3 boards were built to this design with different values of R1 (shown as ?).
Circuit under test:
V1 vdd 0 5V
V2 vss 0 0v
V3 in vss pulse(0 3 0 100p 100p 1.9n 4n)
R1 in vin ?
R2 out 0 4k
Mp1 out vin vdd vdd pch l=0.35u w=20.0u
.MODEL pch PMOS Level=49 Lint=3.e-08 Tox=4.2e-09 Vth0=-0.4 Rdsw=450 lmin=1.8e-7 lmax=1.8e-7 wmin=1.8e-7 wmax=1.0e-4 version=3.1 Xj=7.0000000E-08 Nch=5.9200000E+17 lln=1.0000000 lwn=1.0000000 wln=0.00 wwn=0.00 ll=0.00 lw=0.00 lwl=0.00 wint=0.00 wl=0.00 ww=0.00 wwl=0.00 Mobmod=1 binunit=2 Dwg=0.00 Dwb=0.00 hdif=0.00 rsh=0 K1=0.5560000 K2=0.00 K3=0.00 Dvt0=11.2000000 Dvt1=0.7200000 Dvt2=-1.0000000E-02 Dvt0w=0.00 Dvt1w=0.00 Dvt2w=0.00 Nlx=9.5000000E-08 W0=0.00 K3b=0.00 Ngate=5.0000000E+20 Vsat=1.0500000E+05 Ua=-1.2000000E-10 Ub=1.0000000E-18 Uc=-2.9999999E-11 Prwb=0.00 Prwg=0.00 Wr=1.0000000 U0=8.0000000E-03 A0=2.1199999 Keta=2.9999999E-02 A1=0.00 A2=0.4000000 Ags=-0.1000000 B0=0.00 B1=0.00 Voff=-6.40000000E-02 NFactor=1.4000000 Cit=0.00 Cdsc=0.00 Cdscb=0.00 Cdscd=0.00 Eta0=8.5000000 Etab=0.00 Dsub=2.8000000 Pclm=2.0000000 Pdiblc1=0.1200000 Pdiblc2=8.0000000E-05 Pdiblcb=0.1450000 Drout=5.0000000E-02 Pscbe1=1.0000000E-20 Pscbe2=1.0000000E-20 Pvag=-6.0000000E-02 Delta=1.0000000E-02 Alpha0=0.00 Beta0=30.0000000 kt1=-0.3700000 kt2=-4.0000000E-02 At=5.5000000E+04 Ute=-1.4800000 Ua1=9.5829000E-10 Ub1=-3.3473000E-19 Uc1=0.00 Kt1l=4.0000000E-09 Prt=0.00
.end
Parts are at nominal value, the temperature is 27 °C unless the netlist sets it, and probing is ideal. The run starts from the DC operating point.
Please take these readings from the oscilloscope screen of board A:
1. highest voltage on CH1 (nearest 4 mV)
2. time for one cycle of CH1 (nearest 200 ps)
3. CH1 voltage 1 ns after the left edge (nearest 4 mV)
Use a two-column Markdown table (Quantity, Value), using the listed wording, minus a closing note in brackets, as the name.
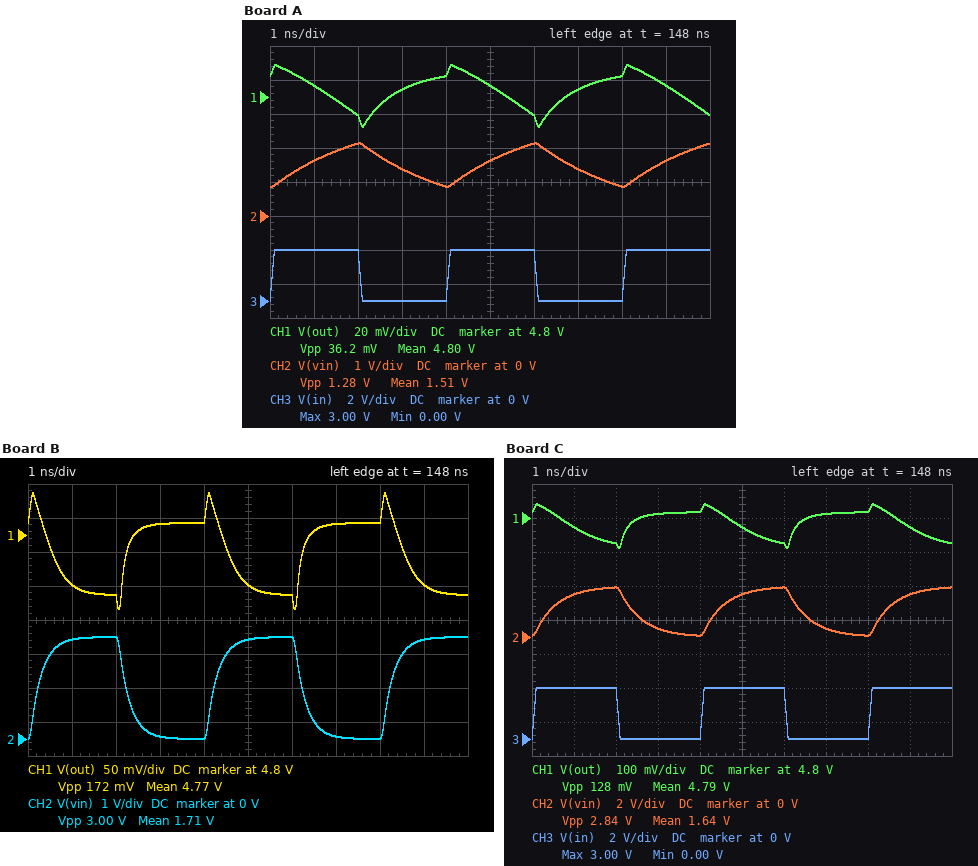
| Quantity | Value |
|---|---|
| highest voltage on CH1 | 4.820 V |
| time for one cycle of CH1 | 4.0 ns |
| CH1 voltage 1 ns after the left edge | 4.808 V |
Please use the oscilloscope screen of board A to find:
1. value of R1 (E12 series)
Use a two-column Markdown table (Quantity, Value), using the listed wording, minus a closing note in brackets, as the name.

| Quantity | Value |
|---|---|
| value of R1 | 33 kΩ |
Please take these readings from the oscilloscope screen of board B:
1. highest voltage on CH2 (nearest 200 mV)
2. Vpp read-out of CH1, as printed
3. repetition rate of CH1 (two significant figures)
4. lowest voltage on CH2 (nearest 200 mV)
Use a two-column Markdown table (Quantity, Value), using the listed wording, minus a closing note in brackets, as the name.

| Quantity | Value |
|---|---|
| highest voltage on CH2 | 3.0 V |
| Vpp read-out of CH1, as printed | 172 mV |
| repetition rate of CH1 | 250 MHz |
| lowest voltage on CH2 | 0 V |
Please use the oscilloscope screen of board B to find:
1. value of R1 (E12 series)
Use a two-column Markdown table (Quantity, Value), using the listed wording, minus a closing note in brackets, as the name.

| Quantity | Value |
|---|---|
| value of R1 | 3.9 kΩ |
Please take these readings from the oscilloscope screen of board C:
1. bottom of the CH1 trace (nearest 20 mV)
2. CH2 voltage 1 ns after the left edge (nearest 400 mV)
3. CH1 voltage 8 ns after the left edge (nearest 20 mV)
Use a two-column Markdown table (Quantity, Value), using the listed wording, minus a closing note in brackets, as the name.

| Quantity | Value |
|---|---|
| bottom of the CH1 trace | 4.72 V |
| CH2 voltage 1 ns after the left edge | 2.4 V |
| CH1 voltage 8 ns after the left edge | 4.82 V |
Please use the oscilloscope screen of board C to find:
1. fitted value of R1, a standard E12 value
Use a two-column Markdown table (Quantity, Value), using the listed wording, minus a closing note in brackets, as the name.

| Quantity | Value |
|---|---|
| fitted value of R1, a standard E12 value | 8.2 kΩ |
